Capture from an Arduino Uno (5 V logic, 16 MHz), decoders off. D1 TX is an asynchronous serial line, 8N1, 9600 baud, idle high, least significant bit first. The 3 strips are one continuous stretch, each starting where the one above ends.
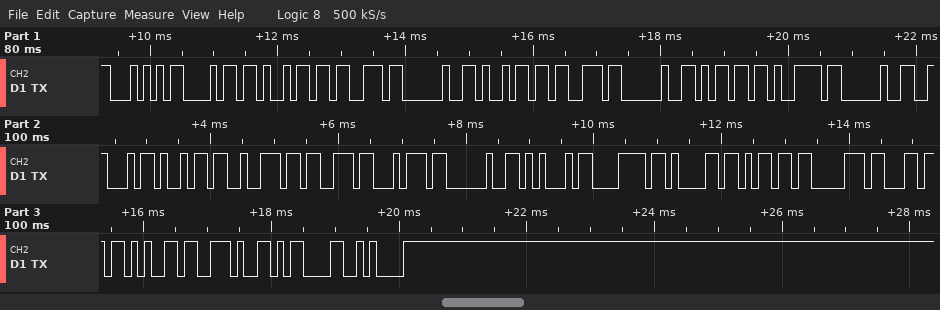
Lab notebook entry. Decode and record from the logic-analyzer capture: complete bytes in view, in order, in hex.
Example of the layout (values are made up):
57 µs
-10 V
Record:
0x54 0x68 0x69 0x73 0x20 0x69 0x73 0x20 0x6D 0x79 0x20 0x46 0x69 0x72 0x73 0x74 0x20 0x45 0x78 0x61 0x6D 0x70 0x6C 0x65 0x2E 0x0D 0x0A
